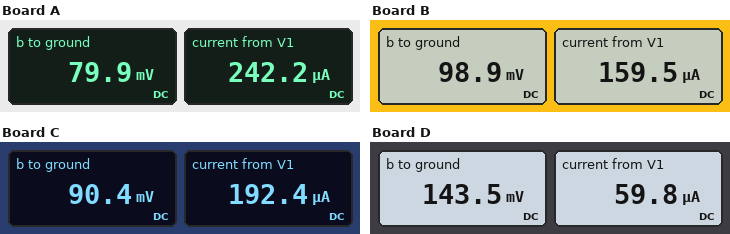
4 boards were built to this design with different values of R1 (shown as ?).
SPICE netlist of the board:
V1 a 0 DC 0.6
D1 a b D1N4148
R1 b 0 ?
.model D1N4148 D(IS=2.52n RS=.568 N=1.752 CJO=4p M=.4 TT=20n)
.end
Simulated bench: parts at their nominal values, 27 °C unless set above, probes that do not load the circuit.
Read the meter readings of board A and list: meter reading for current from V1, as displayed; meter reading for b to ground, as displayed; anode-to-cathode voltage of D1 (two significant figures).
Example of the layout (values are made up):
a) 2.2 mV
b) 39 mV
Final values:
a) 242.2 µA
b) 79.9 mV
c) 520 mV
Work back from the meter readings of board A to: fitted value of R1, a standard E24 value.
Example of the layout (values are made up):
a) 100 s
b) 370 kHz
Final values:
a) 330 Ω
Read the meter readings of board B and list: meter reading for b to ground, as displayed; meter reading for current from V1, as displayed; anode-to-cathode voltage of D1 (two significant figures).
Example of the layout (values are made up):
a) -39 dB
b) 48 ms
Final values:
a) 98.9 mV
b) 159.5 µA
c) 500 mV
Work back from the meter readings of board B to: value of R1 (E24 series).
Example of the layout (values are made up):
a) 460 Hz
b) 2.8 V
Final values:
a) 620 Ω
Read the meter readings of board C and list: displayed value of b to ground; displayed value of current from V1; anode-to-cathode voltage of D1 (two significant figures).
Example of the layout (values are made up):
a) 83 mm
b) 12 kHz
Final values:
a) 90.4 mV
b) 192.4 µA
c) 510 mV
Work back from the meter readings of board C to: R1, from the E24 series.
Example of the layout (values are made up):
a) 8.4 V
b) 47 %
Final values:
a) 470 Ω
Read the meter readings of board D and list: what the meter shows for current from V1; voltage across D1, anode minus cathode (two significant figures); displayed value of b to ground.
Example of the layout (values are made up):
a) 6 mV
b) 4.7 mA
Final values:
a) 59.8 µA
b) 460 mV
c) 143.5 mV
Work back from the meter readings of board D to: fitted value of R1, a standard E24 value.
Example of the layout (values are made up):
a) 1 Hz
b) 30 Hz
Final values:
a) 2.4 kΩ
